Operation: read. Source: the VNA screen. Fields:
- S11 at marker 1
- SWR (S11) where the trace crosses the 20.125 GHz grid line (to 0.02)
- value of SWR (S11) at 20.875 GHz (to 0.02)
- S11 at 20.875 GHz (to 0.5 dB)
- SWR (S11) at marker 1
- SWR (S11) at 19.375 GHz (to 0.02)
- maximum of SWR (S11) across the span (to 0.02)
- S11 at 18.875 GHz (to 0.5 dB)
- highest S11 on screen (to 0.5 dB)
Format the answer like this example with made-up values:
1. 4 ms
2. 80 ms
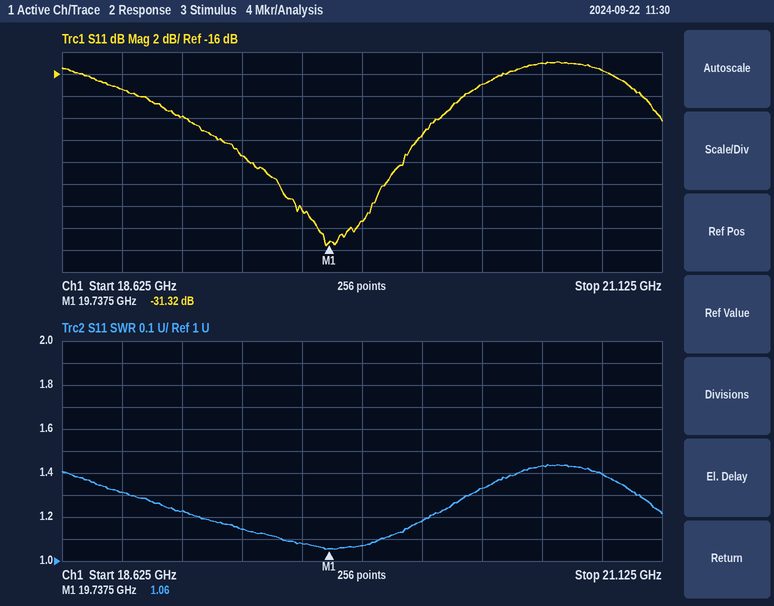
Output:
1. -31.32 dB
2. 1.18
3. 1.40
4. -15.5 dB
5. 1.06
6. 1.14
7. 1.44
8. -17.5 dB
9. -15.0 dB
